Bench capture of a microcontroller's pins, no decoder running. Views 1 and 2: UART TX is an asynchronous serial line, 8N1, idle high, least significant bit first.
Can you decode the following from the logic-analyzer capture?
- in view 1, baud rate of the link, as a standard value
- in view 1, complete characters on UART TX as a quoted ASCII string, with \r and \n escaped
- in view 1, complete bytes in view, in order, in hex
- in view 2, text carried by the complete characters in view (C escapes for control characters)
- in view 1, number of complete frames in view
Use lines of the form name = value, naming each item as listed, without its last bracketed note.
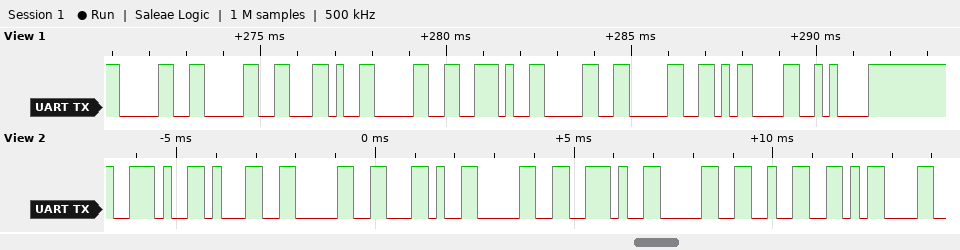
in view 1, baud rate of the link, as a standard value = 4800 baud
in view 1, complete characters on UART TX as a quoted ASCII string, with \r and \n escaped = "00,0.00\r\n"
in view 1, complete bytes in view, in order, in hex = 30 30 2C 30 2E 30 30 0D 0A
in view 2, text carried by the complete characters in view = ".10,0.02\r"
in view 1, number of complete frames in view = 9
